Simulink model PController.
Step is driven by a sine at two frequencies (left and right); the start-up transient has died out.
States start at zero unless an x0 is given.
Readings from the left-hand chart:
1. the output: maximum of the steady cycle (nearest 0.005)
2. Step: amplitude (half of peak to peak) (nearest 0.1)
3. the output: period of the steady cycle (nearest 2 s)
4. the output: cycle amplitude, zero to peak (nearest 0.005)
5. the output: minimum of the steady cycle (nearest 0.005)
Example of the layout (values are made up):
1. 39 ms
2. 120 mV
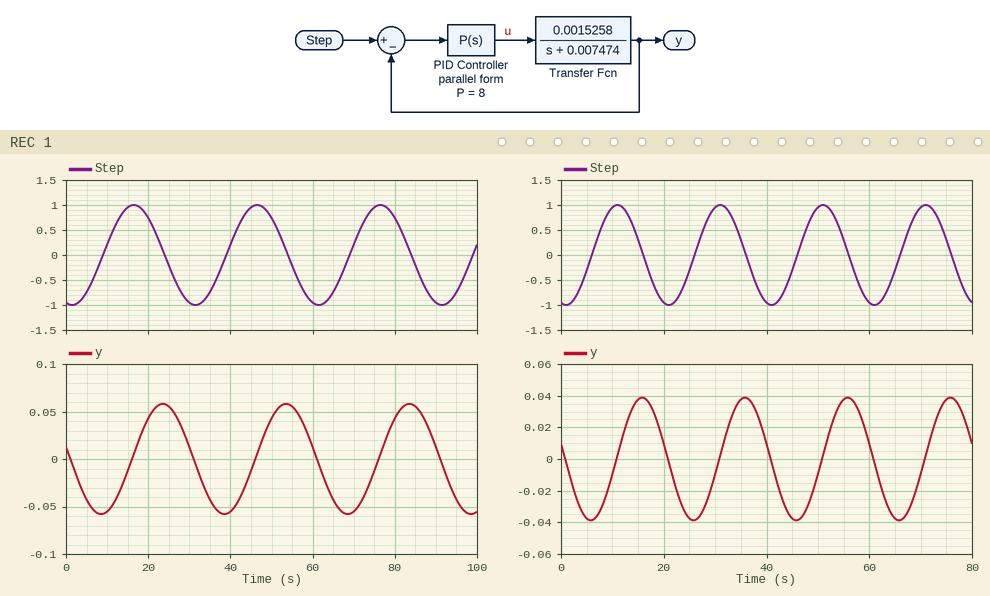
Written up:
1. 0.060
2. 1.0
3. 30 s
4. 0.060
5. -0.060
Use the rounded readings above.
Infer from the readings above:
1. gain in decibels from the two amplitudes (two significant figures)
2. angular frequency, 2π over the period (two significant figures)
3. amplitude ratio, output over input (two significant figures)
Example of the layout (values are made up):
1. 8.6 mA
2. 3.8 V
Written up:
1. -24 dB
2. 0.21 rad/s
3. 0.060
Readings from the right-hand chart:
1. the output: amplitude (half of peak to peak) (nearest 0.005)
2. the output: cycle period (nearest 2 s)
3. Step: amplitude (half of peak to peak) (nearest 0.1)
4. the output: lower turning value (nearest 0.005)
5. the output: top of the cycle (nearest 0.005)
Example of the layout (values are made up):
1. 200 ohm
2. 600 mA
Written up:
1. 0.040
2. 20 s
3. 1.0
4. -0.040
5. 0.040
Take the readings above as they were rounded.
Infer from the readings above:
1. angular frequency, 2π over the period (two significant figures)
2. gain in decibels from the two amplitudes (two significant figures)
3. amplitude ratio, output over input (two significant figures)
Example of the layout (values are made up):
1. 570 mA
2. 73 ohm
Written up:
1. 0.31 rad/s
2. -28 dB
3. 0.040
